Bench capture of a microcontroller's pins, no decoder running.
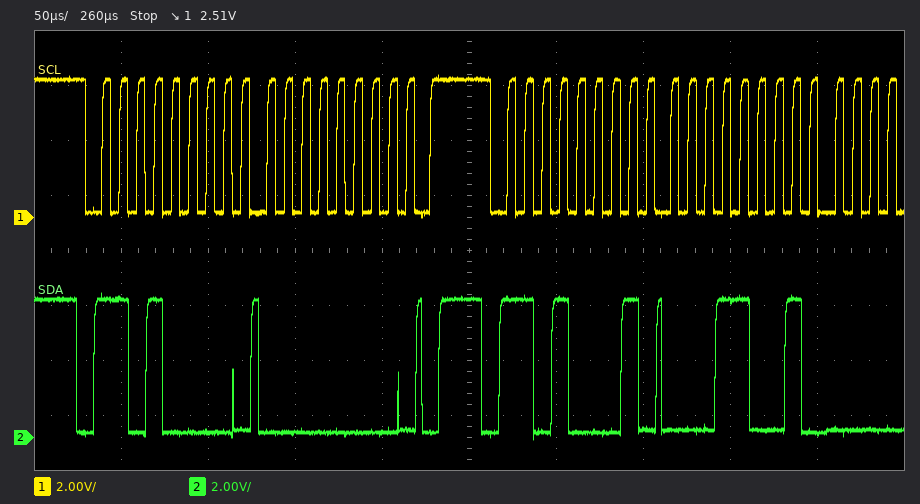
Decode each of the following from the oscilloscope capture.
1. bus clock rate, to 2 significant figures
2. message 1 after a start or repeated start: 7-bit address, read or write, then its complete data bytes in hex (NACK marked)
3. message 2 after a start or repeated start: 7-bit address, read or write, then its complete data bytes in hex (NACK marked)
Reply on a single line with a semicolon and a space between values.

100 kHz; 0x68 write: 00; 0x68 read: 19
